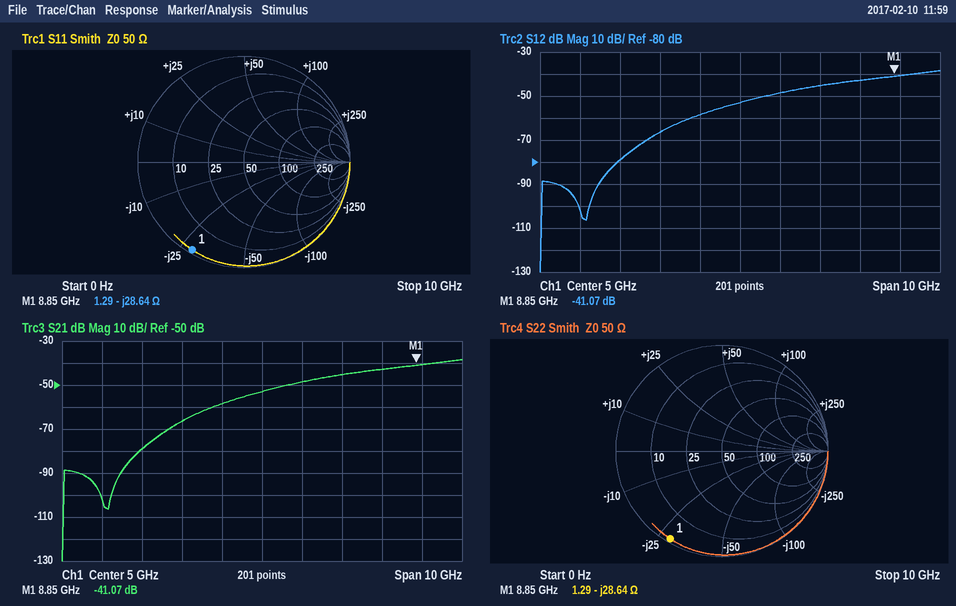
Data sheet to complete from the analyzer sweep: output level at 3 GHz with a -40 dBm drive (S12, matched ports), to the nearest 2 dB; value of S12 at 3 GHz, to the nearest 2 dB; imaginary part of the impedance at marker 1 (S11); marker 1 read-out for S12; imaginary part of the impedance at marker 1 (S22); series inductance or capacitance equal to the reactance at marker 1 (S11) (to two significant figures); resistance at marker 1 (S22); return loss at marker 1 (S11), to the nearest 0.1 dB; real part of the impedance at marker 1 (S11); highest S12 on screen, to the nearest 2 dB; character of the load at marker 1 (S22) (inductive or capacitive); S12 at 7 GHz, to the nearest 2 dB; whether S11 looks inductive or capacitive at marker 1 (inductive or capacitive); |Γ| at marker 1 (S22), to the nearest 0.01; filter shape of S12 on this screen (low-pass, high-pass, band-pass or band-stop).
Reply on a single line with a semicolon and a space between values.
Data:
-106 dBm; -66 dB; -28.64 Ω; -41.07 dB; -28.64 Ω; 630 fF; 1.29 Ω; 0.3 dB; 1.29 Ω; -38 dB; capacitive; -46 dB; capacitive; 0.96; high-pass
